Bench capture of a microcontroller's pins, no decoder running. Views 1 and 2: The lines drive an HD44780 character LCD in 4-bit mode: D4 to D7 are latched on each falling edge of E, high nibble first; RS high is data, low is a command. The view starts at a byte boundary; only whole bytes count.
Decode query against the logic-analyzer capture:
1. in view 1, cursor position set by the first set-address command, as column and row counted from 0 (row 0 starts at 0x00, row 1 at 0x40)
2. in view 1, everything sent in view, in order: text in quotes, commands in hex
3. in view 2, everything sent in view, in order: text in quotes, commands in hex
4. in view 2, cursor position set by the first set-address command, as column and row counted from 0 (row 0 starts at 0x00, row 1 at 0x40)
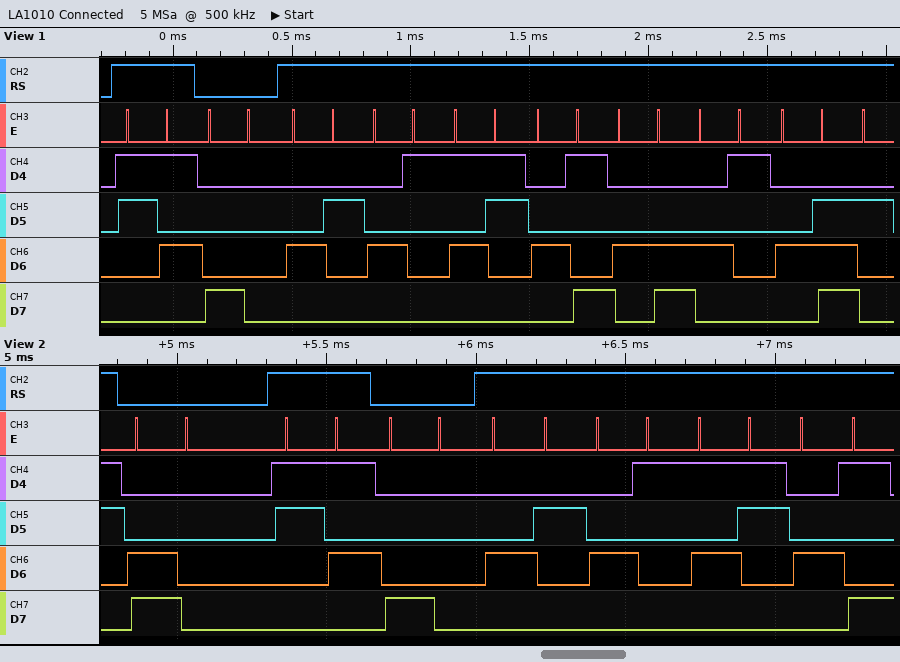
column 0, row 0
"5" 0x80 "BASILAN"
0xC0 "5" 0x80 "BASI"
column 0, row 1
